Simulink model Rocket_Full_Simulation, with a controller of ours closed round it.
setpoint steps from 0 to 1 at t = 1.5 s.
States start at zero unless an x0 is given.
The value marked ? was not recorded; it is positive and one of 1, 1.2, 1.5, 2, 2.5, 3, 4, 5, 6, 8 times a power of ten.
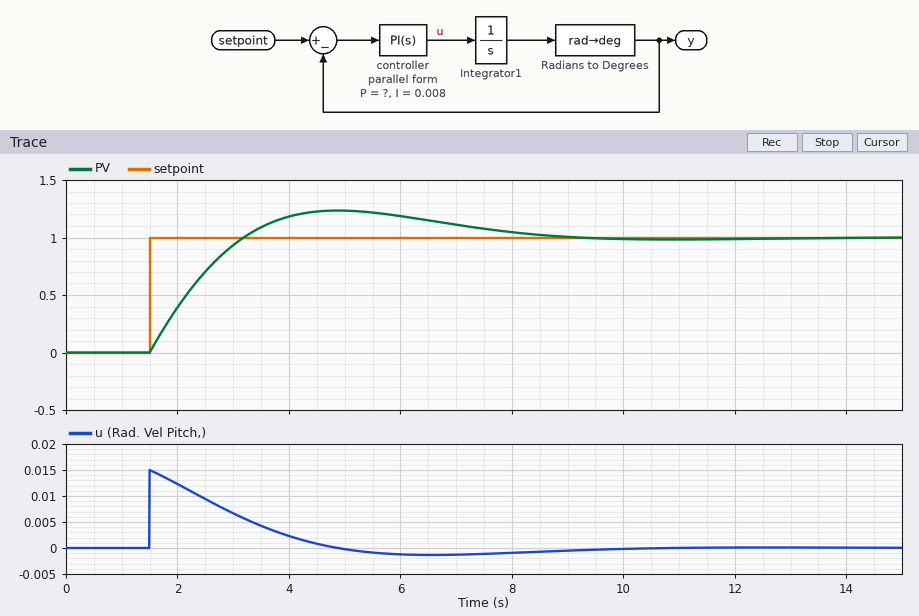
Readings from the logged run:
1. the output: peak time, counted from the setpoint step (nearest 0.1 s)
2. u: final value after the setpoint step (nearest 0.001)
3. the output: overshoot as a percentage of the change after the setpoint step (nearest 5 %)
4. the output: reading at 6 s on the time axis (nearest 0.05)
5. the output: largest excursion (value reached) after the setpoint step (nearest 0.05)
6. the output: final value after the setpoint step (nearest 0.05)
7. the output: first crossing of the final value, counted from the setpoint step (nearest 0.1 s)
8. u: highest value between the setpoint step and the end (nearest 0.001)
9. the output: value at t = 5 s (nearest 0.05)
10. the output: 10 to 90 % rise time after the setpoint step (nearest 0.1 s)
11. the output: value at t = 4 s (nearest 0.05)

3.4 s
0.000
25 %
1.20
1.25
1.00
1.7 s
0.015
1.25
1.3 s
1.20
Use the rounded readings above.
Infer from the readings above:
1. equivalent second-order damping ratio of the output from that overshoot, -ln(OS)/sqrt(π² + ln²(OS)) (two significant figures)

0.40
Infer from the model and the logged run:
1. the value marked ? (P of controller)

0.015
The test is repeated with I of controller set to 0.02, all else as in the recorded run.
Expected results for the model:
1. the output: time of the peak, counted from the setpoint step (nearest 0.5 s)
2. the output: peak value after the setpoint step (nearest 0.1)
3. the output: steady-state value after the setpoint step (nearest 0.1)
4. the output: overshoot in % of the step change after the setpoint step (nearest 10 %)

2.5 s
1.4
1.0
40 %
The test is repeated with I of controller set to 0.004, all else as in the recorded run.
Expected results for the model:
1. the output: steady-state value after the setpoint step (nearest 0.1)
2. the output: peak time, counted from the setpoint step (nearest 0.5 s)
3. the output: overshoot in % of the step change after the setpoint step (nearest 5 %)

1.0
4.5 s
15 %
